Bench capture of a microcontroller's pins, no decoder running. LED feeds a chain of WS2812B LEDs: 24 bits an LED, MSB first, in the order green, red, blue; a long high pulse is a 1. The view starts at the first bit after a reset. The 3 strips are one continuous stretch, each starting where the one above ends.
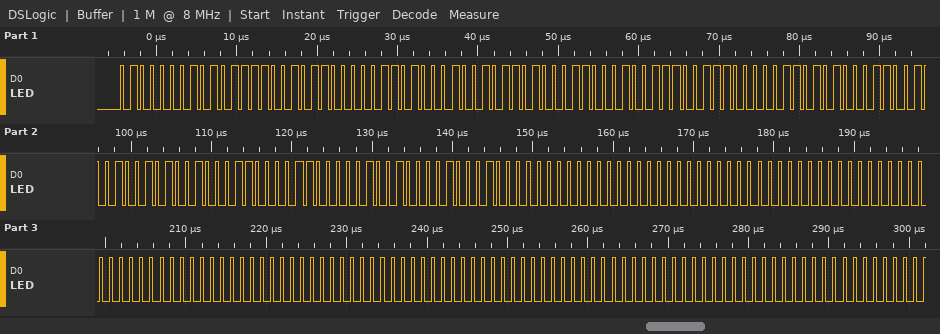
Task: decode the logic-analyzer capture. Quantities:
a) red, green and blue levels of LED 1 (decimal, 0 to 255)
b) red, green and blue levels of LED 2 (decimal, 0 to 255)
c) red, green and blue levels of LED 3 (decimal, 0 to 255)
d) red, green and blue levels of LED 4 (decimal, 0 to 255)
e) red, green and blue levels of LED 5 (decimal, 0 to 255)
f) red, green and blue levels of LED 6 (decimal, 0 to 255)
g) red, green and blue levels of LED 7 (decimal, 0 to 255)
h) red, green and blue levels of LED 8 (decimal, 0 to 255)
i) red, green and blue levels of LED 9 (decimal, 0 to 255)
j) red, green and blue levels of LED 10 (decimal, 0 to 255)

94, 65, 88
75, 52, 70
56, 39, 53
37, 25, 35
18, 12, 17
0, 0, 0
0, 0, 0
0, 0, 0
0, 0, 0
0, 0, 0
